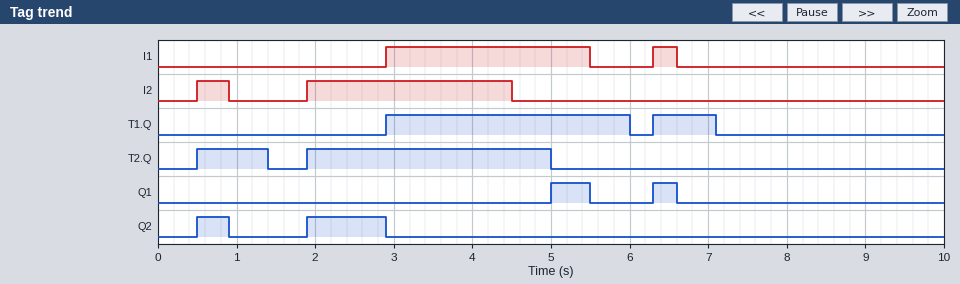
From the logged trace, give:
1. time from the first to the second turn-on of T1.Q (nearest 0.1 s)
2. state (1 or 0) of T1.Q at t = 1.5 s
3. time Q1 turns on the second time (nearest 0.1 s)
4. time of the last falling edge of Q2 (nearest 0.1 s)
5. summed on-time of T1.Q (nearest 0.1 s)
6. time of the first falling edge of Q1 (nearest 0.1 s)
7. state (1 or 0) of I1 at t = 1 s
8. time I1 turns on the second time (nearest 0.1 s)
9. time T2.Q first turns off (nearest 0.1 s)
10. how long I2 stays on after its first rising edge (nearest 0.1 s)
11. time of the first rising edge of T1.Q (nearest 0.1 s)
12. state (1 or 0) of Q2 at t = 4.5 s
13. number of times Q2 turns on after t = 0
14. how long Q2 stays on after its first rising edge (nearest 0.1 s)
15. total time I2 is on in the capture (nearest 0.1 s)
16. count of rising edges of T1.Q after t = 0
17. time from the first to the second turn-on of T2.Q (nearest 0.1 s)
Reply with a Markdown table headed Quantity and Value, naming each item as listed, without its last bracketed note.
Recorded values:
| Quantity | Value |
|---|---|
| time from the first to the second turn-on of T1.Q | 3.4 s |
| state (1 or 0) of T1.Q at t = 1.5 s | 0 |
| time Q1 turns on the second time | 6.3 s |
| time of the last falling edge of Q2 | 2.9 s |
| summed on-time of T1.Q | 3.9 s |
| time of the first falling edge of Q1 | 5.5 s |
| state (1 or 0) of I1 at t = 1 s | 0 |
| time I1 turns on the second time | 6.3 s |
| time T2.Q first turns off | 1.4 s |
| how long I2 stays on after its first rising edge | 0.4 s |
| time of the first rising edge of T1.Q | 2.9 s |
| state (1 or 0) of Q2 at t = 4.5 s | 0 |
| number of times Q2 turns on after t = 0 | 2 |
| how long Q2 stays on after its first rising edge | 0.4 s |
| total time I2 is on in the capture | 3.0 s |
| count of rising edges of T1.Q after t = 0 | 2 |
| time from the first to the second turn-on of T2.Q | 1.4 s |
